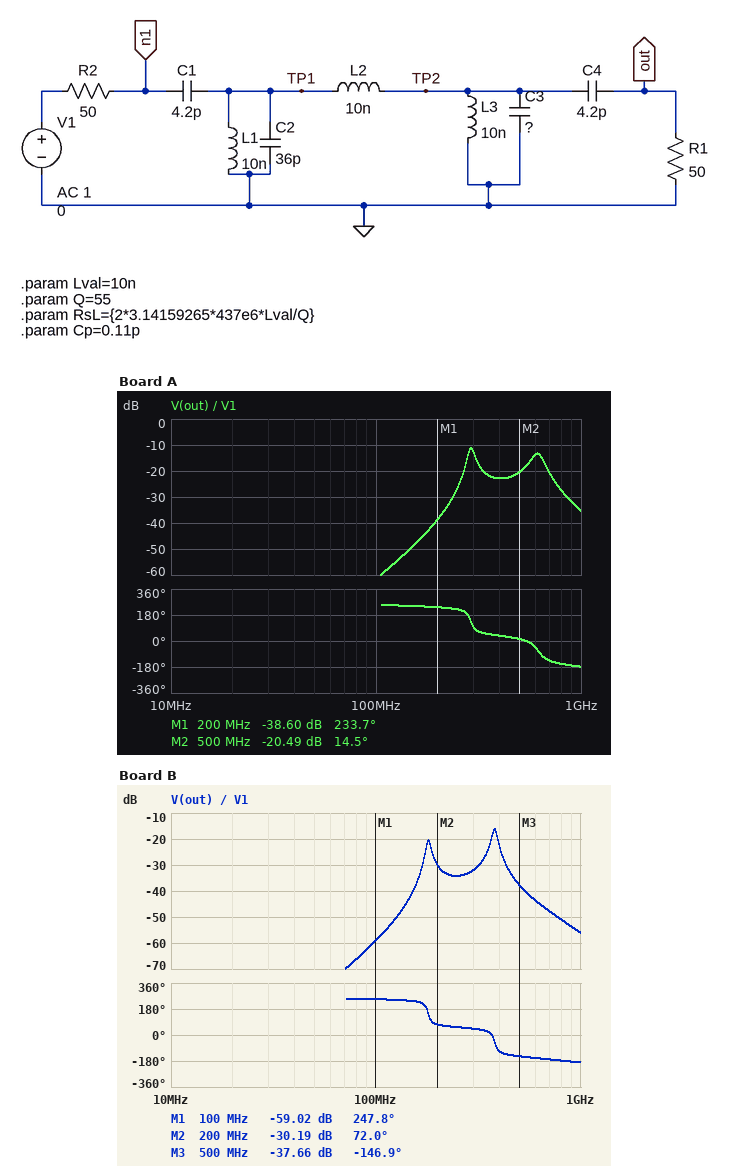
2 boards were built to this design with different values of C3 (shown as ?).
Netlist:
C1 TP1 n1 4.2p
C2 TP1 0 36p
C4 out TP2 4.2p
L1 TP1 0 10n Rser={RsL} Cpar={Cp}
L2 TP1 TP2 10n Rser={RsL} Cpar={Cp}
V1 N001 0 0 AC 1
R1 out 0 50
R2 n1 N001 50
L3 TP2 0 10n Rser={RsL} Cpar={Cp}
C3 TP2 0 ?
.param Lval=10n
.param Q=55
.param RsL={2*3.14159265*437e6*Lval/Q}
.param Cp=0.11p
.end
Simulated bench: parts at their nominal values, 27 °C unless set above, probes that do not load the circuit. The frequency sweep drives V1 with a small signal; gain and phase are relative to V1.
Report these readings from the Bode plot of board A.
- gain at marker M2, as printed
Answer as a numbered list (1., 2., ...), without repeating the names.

1. -20.49 dB
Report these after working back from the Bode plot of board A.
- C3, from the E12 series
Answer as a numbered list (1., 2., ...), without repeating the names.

1. 12 pF
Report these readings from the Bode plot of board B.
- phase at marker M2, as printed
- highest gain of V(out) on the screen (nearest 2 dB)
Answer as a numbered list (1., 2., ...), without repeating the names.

1. 72.0 deg
2. -16 dB
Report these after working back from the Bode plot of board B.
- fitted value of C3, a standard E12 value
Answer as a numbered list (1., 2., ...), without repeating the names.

1. 100 pF
